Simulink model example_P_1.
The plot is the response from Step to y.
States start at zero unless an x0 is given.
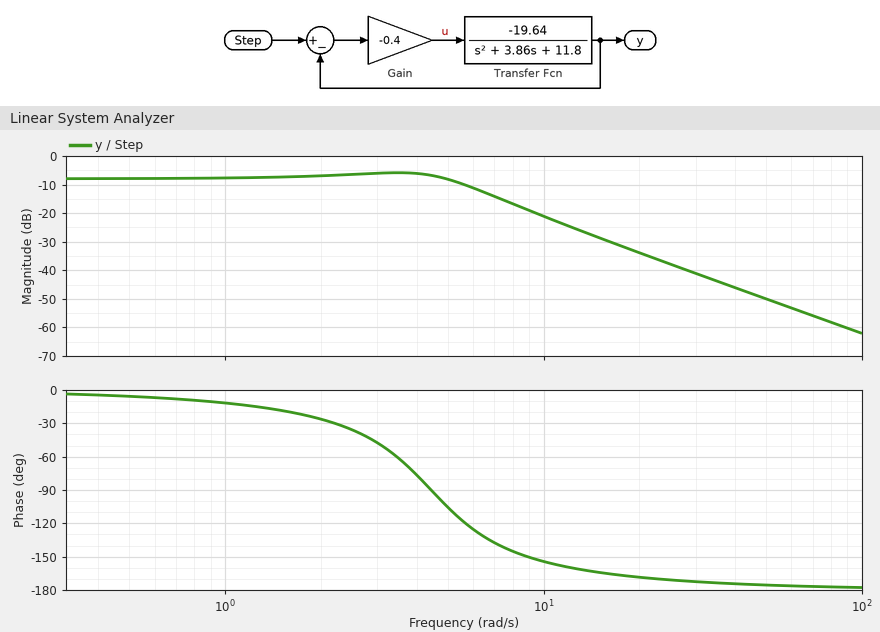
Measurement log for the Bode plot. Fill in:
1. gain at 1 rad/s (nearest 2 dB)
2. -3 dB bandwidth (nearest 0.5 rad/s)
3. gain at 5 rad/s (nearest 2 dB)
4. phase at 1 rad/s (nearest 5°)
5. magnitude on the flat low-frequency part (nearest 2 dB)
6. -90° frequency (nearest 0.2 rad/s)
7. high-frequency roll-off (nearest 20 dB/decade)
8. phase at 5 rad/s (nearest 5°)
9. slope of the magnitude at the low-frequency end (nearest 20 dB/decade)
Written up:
-8 dB
6.0 rad/s
-8 dB
-10°
-8 dB
4.4 rad/s
-40 dB/decade
-105°
0 dB/decade
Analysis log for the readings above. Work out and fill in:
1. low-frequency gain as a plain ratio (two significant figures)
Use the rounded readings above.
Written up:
0.40
